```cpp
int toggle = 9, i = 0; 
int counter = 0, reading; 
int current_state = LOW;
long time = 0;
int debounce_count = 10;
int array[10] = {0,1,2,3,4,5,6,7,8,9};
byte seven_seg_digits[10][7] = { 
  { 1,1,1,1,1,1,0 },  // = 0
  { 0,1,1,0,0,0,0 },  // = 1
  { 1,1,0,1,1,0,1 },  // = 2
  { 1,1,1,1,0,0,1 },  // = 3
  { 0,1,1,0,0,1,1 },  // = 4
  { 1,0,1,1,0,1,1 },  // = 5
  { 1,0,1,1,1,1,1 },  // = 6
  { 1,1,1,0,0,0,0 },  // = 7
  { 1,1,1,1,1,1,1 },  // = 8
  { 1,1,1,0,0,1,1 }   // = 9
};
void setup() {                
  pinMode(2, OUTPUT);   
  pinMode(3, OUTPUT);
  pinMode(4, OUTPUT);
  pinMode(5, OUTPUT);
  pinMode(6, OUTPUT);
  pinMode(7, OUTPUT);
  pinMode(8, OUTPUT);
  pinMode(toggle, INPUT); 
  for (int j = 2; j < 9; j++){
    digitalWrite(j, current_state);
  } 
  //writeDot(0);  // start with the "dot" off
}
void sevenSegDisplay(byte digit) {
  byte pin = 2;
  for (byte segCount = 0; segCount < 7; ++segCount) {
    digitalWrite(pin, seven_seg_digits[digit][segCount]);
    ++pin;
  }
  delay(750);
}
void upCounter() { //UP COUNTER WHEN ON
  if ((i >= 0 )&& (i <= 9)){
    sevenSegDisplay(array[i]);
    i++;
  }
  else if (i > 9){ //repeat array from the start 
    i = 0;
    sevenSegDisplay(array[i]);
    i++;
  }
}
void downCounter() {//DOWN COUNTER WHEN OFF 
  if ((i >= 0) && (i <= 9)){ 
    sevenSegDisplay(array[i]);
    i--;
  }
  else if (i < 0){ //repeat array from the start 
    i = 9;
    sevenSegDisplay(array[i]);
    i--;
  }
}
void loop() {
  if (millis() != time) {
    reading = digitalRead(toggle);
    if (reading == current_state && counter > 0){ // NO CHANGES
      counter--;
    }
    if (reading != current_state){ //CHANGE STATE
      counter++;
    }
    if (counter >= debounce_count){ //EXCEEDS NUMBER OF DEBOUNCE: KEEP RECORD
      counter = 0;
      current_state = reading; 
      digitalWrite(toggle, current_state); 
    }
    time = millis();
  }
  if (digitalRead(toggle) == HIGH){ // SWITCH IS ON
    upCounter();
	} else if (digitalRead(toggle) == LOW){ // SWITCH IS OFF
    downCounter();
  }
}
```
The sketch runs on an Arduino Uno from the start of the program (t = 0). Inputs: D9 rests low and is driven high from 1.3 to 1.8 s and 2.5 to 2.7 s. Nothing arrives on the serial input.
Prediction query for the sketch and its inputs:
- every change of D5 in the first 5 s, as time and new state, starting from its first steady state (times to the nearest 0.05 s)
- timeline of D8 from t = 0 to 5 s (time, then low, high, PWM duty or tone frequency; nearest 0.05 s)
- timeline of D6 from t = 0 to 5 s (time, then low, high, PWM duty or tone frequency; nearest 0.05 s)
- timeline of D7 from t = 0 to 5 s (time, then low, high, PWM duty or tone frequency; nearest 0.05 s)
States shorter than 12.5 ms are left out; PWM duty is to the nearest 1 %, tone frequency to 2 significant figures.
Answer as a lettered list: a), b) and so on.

a) 0 s high; 0.75 s low; 1.5 s high; 2.25 s low; 3 s high; 3.75 s low; 4.5 s high
b) 0 s low; 0.75 s high; 3.75 s low; 4.5 s high
c) 0 s high; 0.75 s low; 1.5 s high; 2.25 s low; 3 s high; 3.75 s low; 4.5 s high
d) 0 s high; 3.75 s low; 4.5 s high
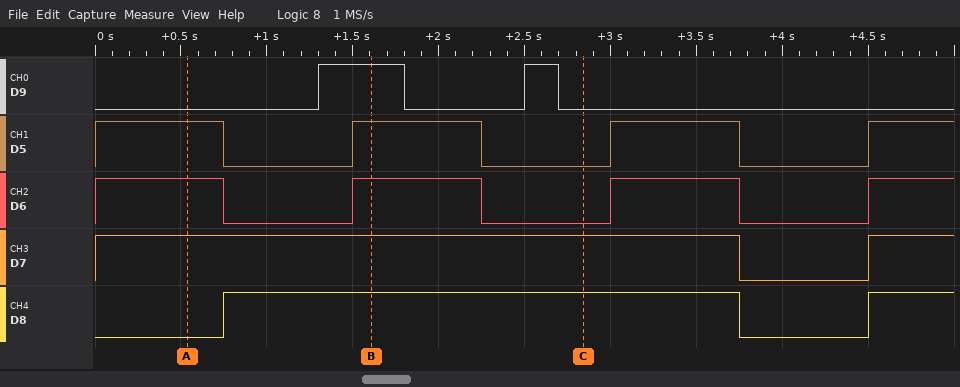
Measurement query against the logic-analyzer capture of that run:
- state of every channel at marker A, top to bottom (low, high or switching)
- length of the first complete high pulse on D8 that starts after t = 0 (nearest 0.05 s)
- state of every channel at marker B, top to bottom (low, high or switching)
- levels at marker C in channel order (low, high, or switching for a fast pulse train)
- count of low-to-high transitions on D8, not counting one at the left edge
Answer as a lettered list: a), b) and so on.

a) D9 low, D5 high, D6 high, D7 high, D8 low
b) 3.00 s
c) D9 high, D5 high, D6 high, D7 high, D8 high
d) D9 low, D5 low, D6 low, D7 high, D8 high
e) 2
